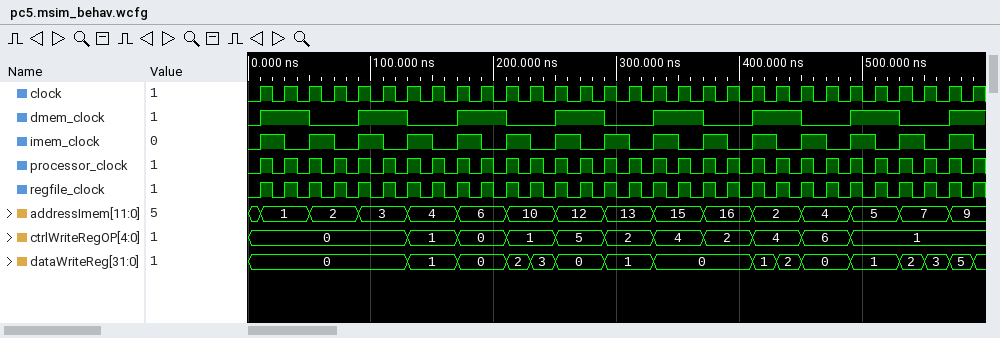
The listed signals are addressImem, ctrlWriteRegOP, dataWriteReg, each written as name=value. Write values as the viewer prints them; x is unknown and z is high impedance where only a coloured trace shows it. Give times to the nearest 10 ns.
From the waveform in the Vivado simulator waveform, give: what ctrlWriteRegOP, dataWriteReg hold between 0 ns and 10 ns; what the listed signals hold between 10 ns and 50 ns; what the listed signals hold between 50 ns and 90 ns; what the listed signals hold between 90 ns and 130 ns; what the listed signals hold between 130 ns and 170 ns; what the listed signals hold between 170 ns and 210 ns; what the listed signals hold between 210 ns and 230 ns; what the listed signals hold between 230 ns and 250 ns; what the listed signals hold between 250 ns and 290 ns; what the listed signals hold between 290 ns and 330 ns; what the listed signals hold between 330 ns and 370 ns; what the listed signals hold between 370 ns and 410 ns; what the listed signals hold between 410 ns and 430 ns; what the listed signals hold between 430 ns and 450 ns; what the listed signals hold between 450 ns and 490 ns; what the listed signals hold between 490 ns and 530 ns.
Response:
ctrlWriteRegOP=0, dataWriteReg=0
addressImem=1, ctrlWriteRegOP=0, dataWriteReg=0
addressImem=2, ctrlWriteRegOP=0, dataWriteReg=0
addressImem=3, ctrlWriteRegOP=0, dataWriteReg=0
addressImem=4, ctrlWriteRegOP=1, dataWriteReg=1
addressImem=6, ctrlWriteRegOP=0, dataWriteReg=0
addressImem=10, ctrlWriteRegOP=1, dataWriteReg=2
addressImem=10, ctrlWriteRegOP=1, dataWriteReg=3
addressImem=12, ctrlWriteRegOP=5, dataWriteReg=0
addressImem=13, ctrlWriteRegOP=2, dataWriteReg=1
addressImem=15, ctrlWriteRegOP=4, dataWriteReg=0
addressImem=16, ctrlWriteRegOP=2, dataWriteReg=0
addressImem=2, ctrlWriteRegOP=4, dataWriteReg=1
addressImem=2, ctrlWriteRegOP=4, dataWriteReg=2
addressImem=4, ctrlWriteRegOP=6, dataWriteReg=0
addressImem=5, ctrlWriteRegOP=1, dataWriteReg=1
